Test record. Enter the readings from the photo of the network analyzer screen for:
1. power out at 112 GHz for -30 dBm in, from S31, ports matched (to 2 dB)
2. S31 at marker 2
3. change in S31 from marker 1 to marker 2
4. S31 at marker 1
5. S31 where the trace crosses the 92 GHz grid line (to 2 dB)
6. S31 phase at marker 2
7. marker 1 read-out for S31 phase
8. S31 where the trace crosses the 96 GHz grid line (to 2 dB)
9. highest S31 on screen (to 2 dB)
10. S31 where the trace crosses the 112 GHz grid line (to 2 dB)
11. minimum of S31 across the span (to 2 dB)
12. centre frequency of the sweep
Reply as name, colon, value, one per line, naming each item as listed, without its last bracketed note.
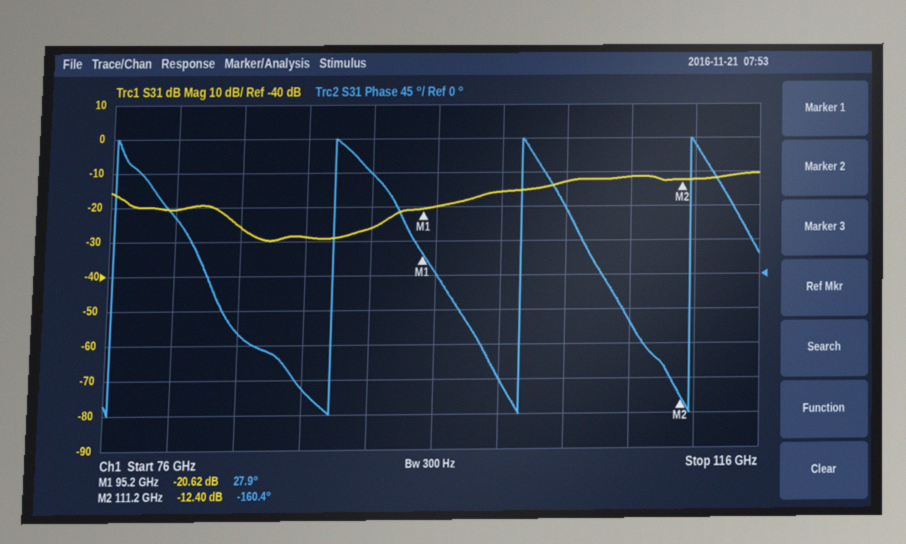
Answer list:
power out at 112 GHz for -30 dBm in, from S31, ports matched: -42 dBm
S31 at marker 2: -12.40 dB
change in S31 from marker 1 to marker 2: 8.22 dB
S31 at marker 1: -20.62 dB
S31 where the trace crosses the 92 GHz grid line: -26 dB
S31 phase at marker 2: -160.4°
marker 1 read-out for S31 phase: 27.9°
S31 where the trace crosses the 96 GHz grid line: -20 dB
highest S31 on screen: -10 dB
S31 where the trace crosses the 112 GHz grid line: -12 dB
minimum of S31 across the span: -30 dB
centre frequency of the sweep: 96 GHz
